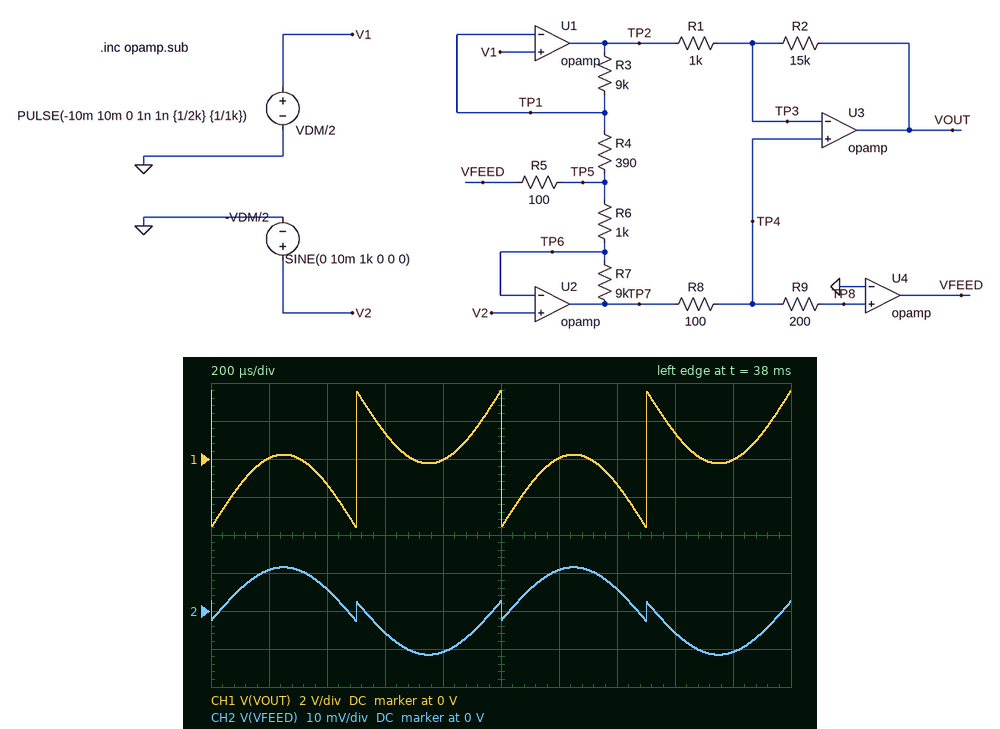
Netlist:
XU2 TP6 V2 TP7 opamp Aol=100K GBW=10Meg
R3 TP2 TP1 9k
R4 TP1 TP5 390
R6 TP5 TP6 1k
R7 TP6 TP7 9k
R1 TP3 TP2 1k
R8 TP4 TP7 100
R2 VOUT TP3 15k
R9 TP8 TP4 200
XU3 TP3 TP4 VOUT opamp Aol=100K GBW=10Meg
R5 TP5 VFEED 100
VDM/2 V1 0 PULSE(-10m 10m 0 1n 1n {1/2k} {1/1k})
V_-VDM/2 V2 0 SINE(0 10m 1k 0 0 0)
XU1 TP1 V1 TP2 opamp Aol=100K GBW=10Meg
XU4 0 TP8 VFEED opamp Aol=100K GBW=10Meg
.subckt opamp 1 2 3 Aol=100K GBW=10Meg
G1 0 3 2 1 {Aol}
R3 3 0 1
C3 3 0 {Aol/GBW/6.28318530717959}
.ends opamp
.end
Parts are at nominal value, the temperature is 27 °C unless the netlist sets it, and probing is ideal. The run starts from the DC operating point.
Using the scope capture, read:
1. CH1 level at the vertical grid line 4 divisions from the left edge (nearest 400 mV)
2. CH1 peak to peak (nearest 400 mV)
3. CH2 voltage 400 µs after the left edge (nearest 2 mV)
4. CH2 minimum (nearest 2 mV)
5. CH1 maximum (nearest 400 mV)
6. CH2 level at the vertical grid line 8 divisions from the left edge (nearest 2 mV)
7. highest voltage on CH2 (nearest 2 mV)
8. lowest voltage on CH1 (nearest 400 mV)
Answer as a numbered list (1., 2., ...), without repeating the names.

1. 0 V
2. 7.2 V
3. 6 mV
4. -12 mV
5. 3.6 V
6. -6 mV
7. 12 mV
8. -3.6 V
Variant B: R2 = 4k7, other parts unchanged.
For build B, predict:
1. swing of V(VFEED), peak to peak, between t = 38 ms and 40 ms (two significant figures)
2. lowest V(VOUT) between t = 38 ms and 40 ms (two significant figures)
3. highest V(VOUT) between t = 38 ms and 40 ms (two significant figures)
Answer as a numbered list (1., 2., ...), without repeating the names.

1. 23 mV
2. -1.1 V
3. 1.1 V
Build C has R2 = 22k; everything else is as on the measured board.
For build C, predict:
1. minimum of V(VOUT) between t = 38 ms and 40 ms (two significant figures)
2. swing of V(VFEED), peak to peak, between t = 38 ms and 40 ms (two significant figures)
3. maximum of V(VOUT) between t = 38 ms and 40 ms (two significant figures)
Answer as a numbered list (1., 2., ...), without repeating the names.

1. -5.3 V
2. 23 mV
3. 5.3 V
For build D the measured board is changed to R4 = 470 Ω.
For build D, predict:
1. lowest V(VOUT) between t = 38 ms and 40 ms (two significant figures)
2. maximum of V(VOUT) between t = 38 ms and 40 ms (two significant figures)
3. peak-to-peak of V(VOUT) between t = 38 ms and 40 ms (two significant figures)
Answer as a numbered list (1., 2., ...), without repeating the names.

1. -3.0 V
2. 3.0 V
3. 6.0 V
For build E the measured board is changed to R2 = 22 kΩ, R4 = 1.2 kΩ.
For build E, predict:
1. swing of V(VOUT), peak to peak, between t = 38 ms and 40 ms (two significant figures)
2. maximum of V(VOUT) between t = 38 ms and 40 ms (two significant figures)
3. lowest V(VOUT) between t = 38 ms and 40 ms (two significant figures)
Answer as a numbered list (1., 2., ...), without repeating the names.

1. 3.7 V
2. 1.9 V
3. -1.9 V
